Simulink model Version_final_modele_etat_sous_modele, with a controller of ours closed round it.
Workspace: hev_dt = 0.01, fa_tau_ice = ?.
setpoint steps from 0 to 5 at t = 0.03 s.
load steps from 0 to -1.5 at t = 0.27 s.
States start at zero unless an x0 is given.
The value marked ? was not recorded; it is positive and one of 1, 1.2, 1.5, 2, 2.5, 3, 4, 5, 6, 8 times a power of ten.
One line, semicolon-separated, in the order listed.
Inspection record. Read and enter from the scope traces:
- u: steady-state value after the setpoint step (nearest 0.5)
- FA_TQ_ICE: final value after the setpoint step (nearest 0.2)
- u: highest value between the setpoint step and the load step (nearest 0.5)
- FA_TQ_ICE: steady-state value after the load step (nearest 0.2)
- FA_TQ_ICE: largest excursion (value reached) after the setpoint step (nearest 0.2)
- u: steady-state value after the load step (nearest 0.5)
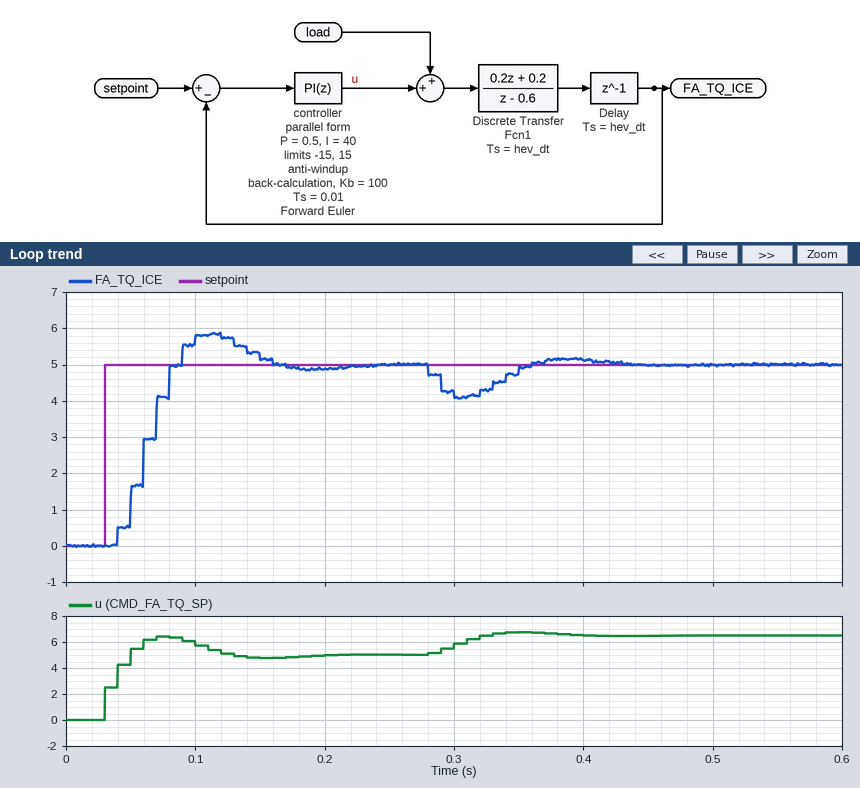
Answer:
5.0; 5.0; 6.5; 5.0; 5.8; 6.5
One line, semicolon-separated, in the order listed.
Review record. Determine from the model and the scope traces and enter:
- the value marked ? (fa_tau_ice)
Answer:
0.02
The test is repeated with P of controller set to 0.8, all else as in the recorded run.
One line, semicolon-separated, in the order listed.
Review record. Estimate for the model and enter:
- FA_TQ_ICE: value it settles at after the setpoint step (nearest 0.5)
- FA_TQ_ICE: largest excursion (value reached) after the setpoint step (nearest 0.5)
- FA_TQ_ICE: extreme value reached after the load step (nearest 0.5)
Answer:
5.0; 5.5; 4.0
